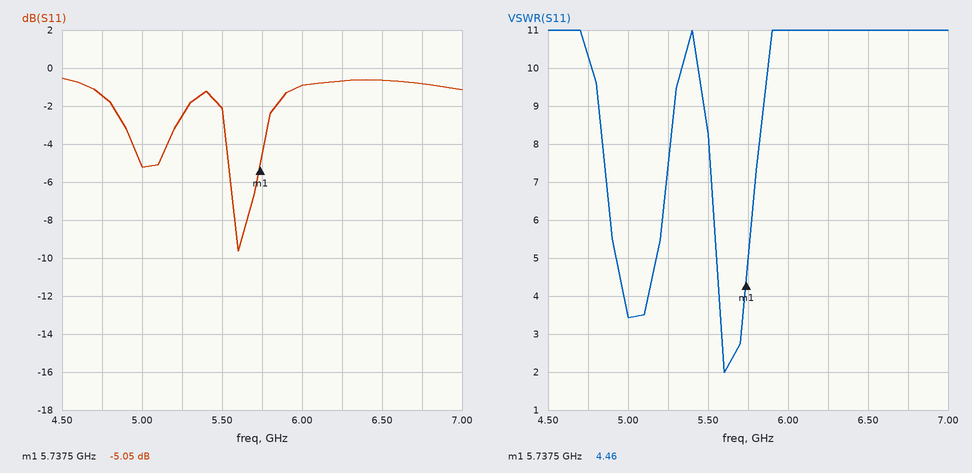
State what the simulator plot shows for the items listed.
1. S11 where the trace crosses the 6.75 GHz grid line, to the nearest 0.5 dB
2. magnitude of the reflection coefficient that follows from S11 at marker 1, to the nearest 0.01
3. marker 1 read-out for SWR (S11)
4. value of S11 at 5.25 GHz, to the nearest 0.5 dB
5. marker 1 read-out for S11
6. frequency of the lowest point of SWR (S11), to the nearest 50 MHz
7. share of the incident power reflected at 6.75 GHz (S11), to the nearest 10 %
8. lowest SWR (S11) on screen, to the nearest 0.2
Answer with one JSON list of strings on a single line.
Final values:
["-1.0 dB", "0.56", "4.46", "-2.5 dB", "-5.05 dB", "5.60 GHz", "80 %", "2.0"]
